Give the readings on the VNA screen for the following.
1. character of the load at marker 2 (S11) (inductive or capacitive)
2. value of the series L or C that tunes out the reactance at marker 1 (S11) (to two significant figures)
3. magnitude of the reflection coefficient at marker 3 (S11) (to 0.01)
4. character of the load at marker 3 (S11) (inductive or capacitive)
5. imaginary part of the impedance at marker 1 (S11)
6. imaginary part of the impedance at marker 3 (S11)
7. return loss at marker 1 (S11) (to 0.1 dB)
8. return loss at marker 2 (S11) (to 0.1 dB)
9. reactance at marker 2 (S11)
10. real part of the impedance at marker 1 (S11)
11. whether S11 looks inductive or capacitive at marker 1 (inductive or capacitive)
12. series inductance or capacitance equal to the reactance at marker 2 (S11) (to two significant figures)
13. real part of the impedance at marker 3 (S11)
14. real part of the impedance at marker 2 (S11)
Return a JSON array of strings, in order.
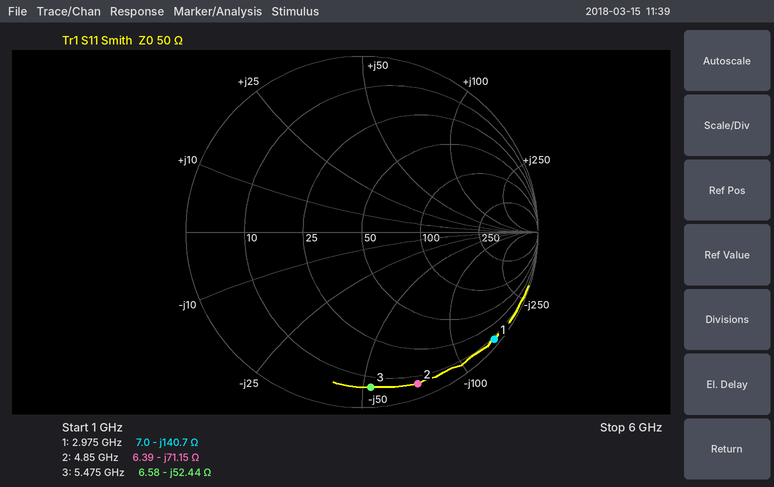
["capacitive", "7.5 nH", "0.88", "capacitive", "-140.7 Ω", "-52.44 Ω", "0.3 dB", "0.7 dB", "-71.15 Ω", "7.0 Ω", "capacitive", "460 fF", "6.58 Ω", "6.39 Ω"]
